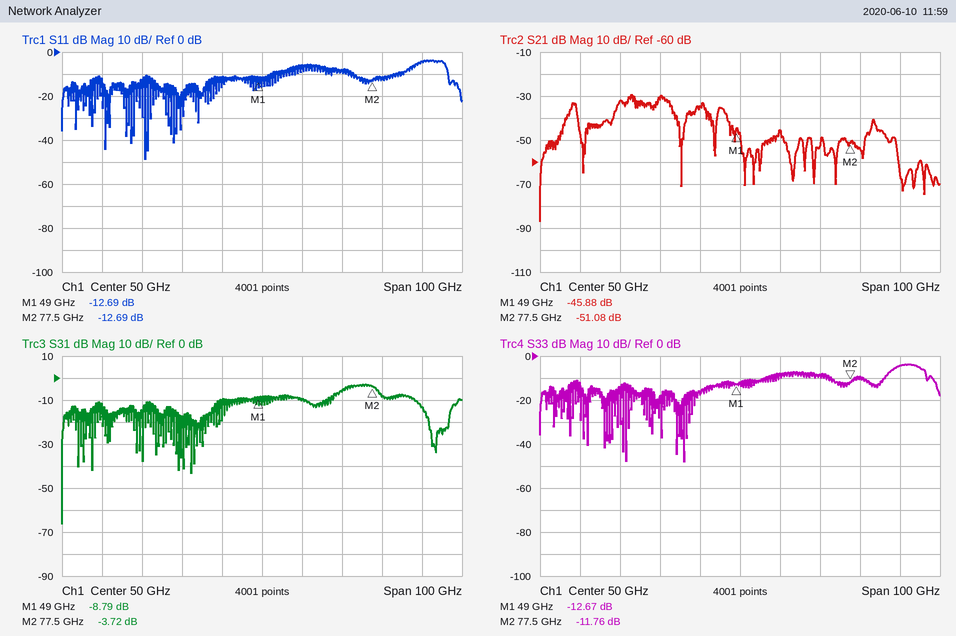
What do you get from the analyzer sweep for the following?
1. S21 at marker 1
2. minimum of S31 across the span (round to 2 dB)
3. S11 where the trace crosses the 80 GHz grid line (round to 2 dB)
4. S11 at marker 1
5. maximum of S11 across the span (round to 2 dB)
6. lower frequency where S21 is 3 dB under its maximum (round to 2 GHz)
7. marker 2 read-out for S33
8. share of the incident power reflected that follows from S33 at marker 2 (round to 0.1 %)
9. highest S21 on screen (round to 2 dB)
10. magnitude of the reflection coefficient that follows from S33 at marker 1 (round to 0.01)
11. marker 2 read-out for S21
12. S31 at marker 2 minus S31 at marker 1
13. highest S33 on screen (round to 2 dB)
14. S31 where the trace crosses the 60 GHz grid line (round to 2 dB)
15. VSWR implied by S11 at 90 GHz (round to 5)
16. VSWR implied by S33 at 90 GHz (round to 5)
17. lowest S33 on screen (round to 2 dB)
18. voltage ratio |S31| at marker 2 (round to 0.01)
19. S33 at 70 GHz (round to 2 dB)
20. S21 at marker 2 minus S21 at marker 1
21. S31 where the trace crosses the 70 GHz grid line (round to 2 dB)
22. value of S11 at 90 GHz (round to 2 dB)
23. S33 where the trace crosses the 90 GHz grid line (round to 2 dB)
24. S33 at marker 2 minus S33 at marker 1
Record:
-45.88 dB
-66 dB
-12 dB
-12.69 dB
-4 dB
22 GHz
-11.76 dB
6.7 %
-30 dB
0.23
-51.08 dB
5.07 dB
-4 dB
-10 dB
5
5
-48 dB
0.65
-8 dB
-5.20 dB
-6 dB
-4 dB
-4 dB
0.91 dB
